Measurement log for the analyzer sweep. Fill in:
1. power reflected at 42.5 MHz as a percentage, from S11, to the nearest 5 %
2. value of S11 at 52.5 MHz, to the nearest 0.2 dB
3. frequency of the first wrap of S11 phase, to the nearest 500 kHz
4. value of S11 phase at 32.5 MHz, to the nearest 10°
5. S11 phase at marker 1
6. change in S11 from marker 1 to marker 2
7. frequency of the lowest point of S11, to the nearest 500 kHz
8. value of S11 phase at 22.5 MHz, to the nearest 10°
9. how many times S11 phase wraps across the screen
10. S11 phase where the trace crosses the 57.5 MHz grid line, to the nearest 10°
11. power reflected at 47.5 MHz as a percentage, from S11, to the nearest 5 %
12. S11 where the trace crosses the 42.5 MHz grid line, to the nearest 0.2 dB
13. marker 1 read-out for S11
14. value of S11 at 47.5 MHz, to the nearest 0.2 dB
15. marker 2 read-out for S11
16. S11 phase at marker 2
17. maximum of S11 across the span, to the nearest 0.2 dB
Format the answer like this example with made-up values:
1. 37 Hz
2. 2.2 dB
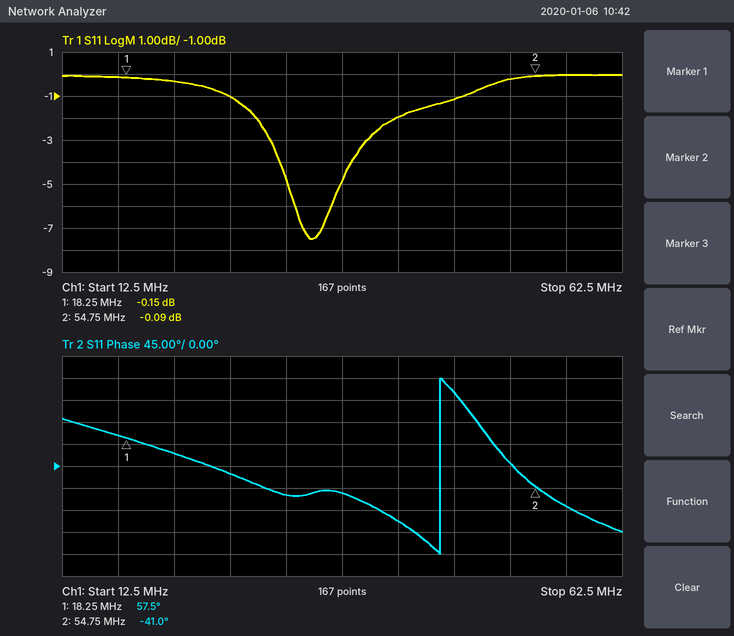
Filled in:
1. 65 %
2. -0.2 dB
3. 46.0 MHz
4. -60°
5. 57.5°
6. 0.06 dB
7. 34.5 MHz
8. 30°
9. 1
10. -80°
11. 75 %
12. -2.0 dB
13. -0.15 dB
14. -1.2 dB
15. -0.09 dB
16. -41.0°
17. 0.0 dB
